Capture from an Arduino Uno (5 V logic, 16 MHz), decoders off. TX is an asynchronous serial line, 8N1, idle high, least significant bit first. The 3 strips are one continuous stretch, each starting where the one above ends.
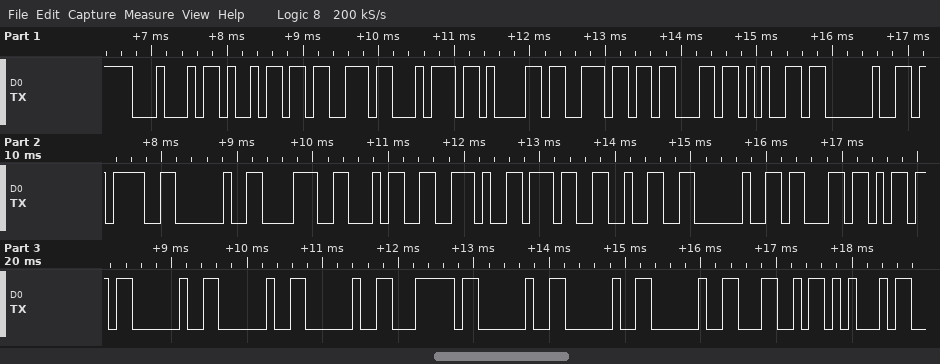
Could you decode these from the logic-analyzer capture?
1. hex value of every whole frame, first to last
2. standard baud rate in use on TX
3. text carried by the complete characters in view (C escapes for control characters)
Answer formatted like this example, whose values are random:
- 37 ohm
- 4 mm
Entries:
- 44 69 73 74 61 6E 63 65 20 3D 20 38 34 2E 37 32 20 63 6D 20 20 20 7C 20 20 20 4C 45
- 9600 baud
- "Distance = 84.72 cm   |   LE"
